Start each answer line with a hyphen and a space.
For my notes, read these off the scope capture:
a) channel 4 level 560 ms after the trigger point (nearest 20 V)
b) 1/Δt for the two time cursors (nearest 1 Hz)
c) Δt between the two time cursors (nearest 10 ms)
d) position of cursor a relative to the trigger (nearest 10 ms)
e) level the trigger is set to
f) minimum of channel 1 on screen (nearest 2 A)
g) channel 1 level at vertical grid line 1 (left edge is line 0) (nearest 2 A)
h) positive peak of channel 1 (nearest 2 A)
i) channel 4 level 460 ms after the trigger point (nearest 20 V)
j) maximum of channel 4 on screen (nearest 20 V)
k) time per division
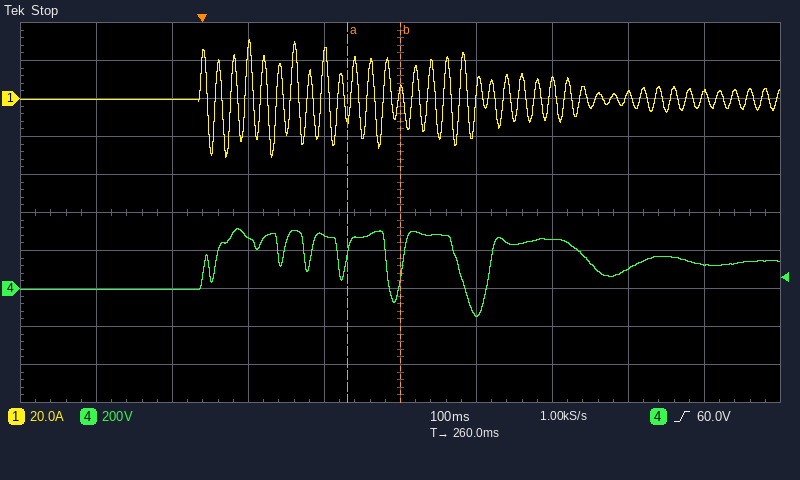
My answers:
- 100 V
- 14 Hz
- 70 ms
- +190 ms
- 60.0 V
- -32 A
- 0 A
- 32 A
- 260 V
- 320 V
- 100 ms
